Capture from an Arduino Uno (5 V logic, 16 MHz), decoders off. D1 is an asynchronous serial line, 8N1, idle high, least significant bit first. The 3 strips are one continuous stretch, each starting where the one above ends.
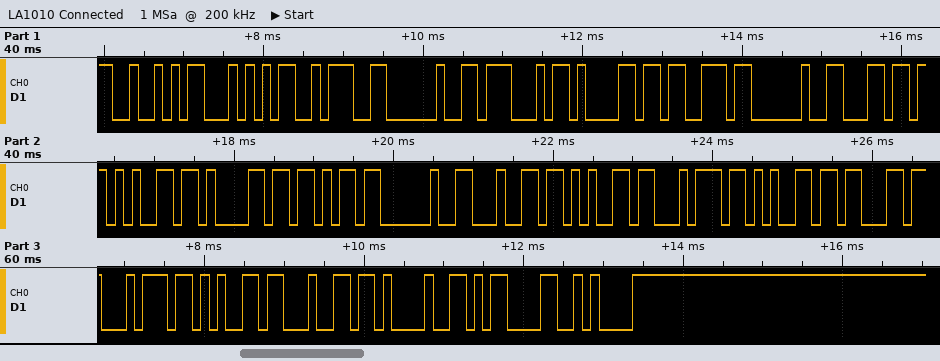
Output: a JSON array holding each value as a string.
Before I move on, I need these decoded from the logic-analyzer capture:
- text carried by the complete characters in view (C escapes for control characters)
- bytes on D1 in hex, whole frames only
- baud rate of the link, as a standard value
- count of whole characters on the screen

["\"RT: Gas leak detected!\\r\\n\"", "52 54 3A 20 47 61 73 20 6C 65 61 6B 20 64 65 74 65 63 74 65 64 21 0D 0A", "9600 baud", "24"]
